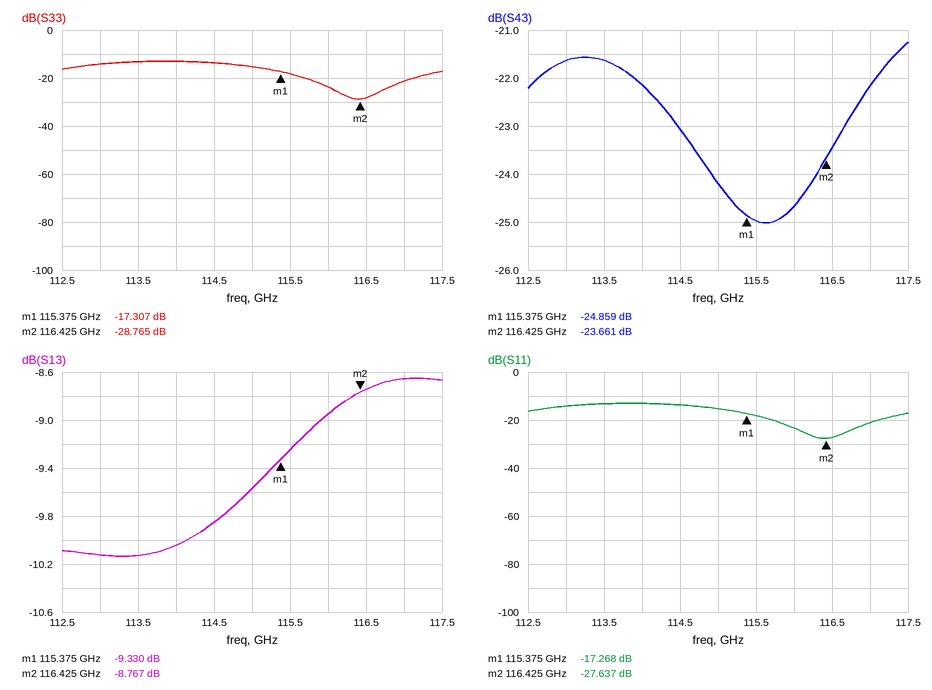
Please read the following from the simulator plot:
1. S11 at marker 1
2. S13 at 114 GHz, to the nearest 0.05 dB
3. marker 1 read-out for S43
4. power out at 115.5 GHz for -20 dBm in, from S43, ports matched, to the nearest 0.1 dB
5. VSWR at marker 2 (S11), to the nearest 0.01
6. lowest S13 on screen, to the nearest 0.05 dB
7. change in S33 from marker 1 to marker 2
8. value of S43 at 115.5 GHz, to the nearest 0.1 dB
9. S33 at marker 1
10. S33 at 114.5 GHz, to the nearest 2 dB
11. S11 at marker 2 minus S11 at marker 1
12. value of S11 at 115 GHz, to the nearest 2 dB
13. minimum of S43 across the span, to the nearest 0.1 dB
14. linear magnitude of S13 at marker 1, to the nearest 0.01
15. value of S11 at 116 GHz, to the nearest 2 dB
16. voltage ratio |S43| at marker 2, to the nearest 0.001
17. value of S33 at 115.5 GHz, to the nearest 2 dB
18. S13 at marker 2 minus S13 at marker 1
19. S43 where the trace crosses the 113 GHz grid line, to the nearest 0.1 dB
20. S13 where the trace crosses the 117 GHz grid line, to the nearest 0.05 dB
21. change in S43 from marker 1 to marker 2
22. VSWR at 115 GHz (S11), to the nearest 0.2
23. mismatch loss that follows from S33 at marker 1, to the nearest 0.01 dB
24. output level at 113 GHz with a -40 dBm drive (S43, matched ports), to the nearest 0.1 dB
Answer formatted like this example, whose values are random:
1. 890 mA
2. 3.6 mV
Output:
1. -17.268 dB
2. -10.05 dB
3. -24.859 dB
4. -45.0 dBm
5. 1.09
6. -10.15 dB
7. -11.458 dB
8. -25.0 dB
9. -17.307 dB
10. -14 dB
11. -10.369 dB
12. -16 dB
13. -25.0 dB
14. 0.34
15. -24 dB
16. 0.066
17. -18 dB
18. 0.563 dB
19. -21.6 dB
20. -8.65 dB
21. 1.198 dB
22. 1.4
23. 0.08 dB
24. -61.6 dBm
